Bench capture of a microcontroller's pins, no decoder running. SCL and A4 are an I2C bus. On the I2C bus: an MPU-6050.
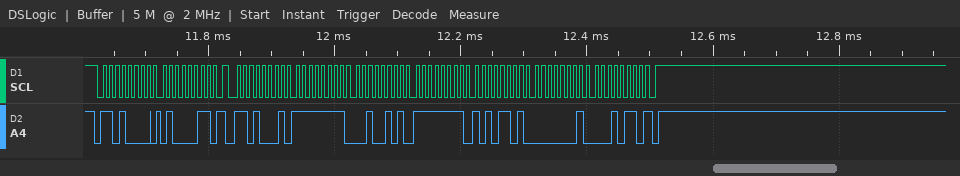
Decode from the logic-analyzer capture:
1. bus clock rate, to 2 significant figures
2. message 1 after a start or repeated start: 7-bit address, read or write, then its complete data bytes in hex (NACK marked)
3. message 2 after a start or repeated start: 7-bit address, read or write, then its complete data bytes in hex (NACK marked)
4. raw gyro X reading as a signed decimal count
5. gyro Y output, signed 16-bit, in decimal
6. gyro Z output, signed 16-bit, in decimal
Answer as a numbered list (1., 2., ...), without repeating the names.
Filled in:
1. 100 kHz
2. 0x68 write: 43
3. 0x68 read: FF 25 FF AD 01 16 NACK
4. -219
5. -83
6. 278
